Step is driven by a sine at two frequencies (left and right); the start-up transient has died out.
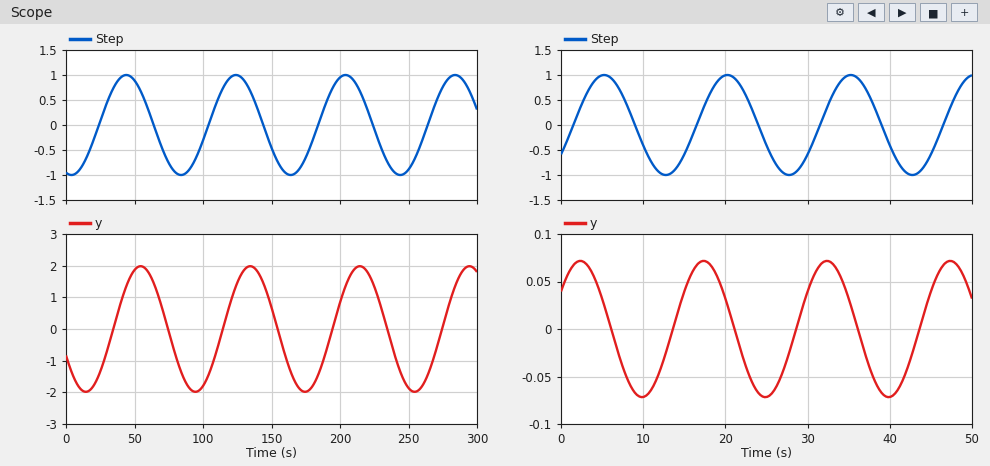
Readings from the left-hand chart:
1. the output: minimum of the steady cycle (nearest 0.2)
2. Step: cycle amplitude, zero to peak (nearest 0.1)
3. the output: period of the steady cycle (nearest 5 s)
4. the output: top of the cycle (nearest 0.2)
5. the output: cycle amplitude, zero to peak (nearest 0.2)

-2.0
1.0
80 s
2.0
2.0
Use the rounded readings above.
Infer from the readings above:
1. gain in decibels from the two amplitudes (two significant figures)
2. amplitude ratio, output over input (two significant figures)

6.0 dB
2.0
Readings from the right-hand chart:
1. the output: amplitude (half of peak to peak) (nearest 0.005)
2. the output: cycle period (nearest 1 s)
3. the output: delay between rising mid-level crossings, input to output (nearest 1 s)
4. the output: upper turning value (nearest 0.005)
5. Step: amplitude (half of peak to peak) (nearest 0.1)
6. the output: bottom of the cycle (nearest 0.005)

0.070
15 s
12 s
0.070
1.0
-0.070
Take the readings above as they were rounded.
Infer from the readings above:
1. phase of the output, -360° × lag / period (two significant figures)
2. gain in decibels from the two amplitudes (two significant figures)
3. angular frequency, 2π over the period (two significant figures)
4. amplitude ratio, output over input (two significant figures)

-290°
-23 dB
0.42 rad/s
0.070
